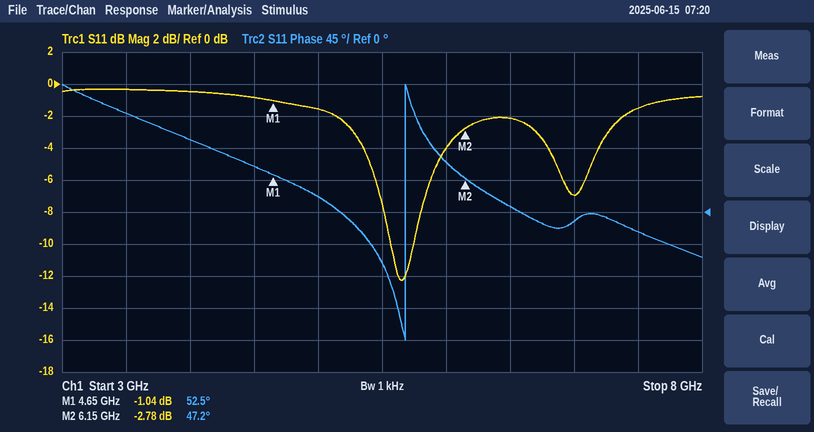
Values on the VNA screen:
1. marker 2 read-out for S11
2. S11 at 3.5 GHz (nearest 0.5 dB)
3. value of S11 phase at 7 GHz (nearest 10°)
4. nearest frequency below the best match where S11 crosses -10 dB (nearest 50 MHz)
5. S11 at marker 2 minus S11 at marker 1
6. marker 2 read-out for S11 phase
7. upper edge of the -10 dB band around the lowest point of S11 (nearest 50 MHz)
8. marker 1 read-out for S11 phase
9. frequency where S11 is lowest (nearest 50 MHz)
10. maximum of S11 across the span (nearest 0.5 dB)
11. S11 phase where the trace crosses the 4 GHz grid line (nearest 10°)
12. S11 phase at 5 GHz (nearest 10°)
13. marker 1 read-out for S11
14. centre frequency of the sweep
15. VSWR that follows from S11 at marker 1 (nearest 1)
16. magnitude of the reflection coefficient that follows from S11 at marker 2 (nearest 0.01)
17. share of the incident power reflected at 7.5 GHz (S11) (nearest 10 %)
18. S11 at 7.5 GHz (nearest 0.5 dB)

-2.78 dB
-0.5 dB
-10°
5.55 GHz
-1.74 dB
47.2°
5.75 GHz
52.5°
5.65 GHz
-0.5 dB
100°
20°
-1.04 dB
5.5 GHz
17
0.73
70 %
-1.5 dB
